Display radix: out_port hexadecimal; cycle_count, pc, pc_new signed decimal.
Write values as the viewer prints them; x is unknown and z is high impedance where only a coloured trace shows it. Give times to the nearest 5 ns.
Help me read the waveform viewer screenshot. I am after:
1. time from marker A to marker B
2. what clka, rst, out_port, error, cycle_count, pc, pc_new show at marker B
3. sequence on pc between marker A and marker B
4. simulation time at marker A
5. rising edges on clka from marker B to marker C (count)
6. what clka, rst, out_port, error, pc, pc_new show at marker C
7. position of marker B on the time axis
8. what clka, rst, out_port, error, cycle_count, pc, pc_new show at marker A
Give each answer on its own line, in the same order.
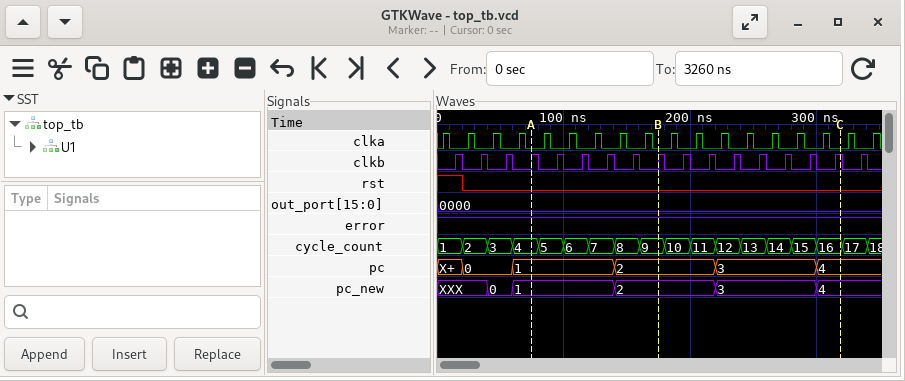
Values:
100 ns
clka=0, rst=0, out_port=0000, error=1, cycle_count=9, pc=2, pc_new=2
1, 2
75 ns
7
clka=0, rst=0, out_port=0000, error=1, pc=4, pc_new=4
175 ns
clka=0, rst=0, out_port=0000, error=1, cycle_count=4, pc=1, pc_new=1
